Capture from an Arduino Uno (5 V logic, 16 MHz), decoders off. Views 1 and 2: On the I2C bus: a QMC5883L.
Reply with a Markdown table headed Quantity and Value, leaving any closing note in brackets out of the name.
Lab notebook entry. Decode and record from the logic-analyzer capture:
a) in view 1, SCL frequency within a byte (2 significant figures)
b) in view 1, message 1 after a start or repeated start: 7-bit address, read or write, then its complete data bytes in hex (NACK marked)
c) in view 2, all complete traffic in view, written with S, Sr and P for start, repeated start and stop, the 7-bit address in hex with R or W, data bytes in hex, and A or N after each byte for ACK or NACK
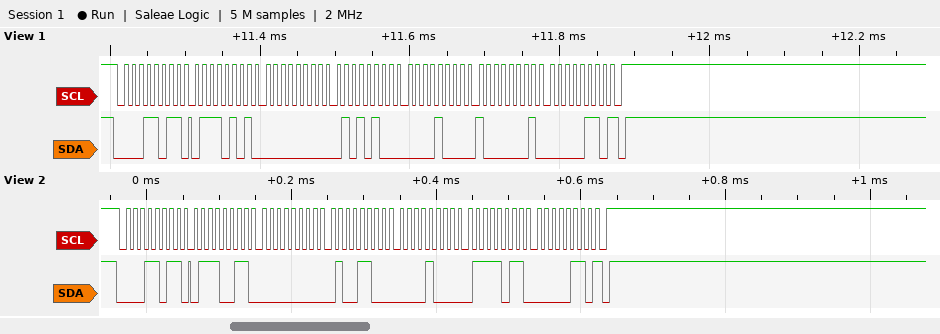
| Quantity | Value |
|---|---|
| in view 1, SCL frequency within a byte | 100 kHz |
| in view 1, message 1 after a start or repeated start: 7-bit address, read or write, then its complete data bytes in hex | 0x0D read: 75 00 54 08 81 06 NACK |
| in view 2, all complete traffic in view, written with S, Sr and P for start, repeated start and stop, the 7-bit address in hex with R or W, data bytes in hex, and A or N after each byte for ACK or NACK | S 0DR A 73 A 00 A 4C A 08 A 7B A 06 N P |
